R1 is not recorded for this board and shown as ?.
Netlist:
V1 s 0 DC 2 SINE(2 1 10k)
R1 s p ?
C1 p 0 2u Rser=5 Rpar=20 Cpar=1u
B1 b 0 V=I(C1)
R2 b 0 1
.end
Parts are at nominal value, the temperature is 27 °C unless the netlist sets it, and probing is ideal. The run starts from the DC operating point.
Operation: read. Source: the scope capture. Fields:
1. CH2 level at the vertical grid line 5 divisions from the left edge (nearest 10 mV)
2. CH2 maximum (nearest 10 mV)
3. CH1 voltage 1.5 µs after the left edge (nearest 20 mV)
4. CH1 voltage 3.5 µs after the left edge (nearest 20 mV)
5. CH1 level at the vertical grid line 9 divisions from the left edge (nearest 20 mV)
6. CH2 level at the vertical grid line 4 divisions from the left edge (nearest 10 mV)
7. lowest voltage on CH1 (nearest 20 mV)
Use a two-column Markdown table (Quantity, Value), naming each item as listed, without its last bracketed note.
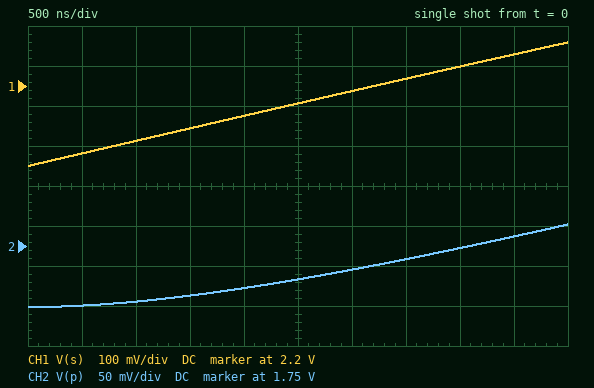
| Quantity | Value |
|---|---|
| CH2 level at the vertical grid line 5 divisions from the left edge | 1.71 V |
| CH2 maximum | 1.78 V |
| CH1 voltage 1.5 µs after the left edge | 2.10 V |
| CH1 voltage 3.5 µs after the left edge | 2.22 V |
| CH1 level at the vertical grid line 9 divisions from the left edge | 2.28 V |
| CH2 level at the vertical grid line 4 divisions from the left edge | 1.70 V |
| lowest voltage on CH1 | 2.00 V |
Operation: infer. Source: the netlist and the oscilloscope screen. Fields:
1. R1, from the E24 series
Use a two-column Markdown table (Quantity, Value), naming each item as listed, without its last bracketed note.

| Quantity | Value |
|---|---|
| R1, from the E24 series | 3.9 Ω |
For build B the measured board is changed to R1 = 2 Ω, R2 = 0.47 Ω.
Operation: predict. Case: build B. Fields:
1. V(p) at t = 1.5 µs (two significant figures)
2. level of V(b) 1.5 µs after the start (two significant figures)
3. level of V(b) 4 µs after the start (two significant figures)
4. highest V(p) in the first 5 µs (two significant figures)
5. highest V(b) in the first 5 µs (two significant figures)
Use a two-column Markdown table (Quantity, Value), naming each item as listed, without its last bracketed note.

| Quantity | Value |
|---|---|
| V(p) at t = 1.5 µs | 1.8 V |
| level of V(b) 1.5 µs after the start | 4.8 mV |
| level of V(b) 4 µs after the start | 20 mV |
| highest V(p) in the first 5 µs | 2.0 V |
| highest V(b) in the first 5 µs | 26 mV |
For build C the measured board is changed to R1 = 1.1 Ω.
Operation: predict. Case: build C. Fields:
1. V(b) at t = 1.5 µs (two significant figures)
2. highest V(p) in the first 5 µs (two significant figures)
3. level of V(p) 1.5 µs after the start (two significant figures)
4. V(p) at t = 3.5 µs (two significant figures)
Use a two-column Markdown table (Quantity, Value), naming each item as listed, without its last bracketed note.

| Quantity | Value |
|---|---|
| V(b) at t = 1.5 µs | 7.4 mV |
| highest V(p) in the first 5 µs | 2.1 V |
| level of V(p) 1.5 µs after the start | 1.9 V |
| V(p) at t = 3.5 µs | 2.0 V |
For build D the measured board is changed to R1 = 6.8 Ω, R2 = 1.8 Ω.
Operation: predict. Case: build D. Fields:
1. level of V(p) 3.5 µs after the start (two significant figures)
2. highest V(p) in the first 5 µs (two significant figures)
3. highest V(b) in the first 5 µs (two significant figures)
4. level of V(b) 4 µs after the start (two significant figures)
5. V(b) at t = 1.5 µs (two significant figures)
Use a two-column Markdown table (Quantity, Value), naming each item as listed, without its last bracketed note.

| Quantity | Value |
|---|---|
| level of V(p) 3.5 µs after the start | 1.5 V |
| highest V(p) in the first 5 µs | 1.6 V |
| highest V(b) in the first 5 µs | 11 mV |
| level of V(b) 4 µs after the start | 8.2 mV |
| V(b) at t = 1.5 µs | 1.6 mV |
